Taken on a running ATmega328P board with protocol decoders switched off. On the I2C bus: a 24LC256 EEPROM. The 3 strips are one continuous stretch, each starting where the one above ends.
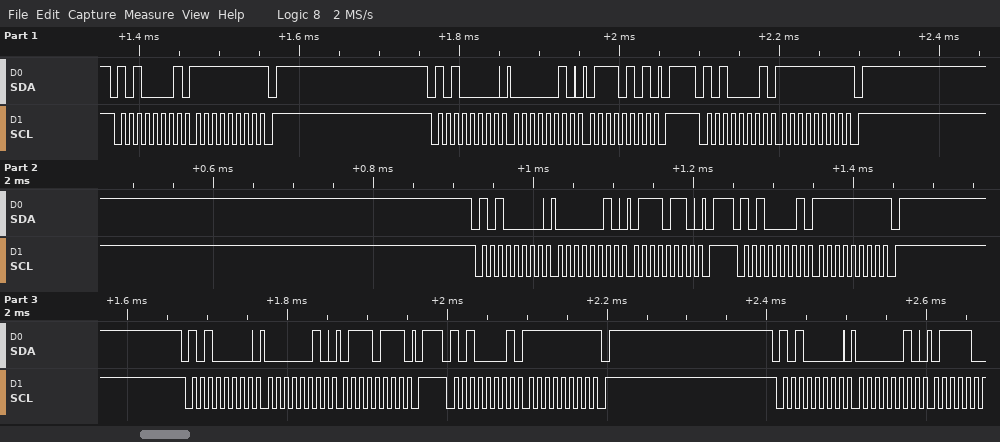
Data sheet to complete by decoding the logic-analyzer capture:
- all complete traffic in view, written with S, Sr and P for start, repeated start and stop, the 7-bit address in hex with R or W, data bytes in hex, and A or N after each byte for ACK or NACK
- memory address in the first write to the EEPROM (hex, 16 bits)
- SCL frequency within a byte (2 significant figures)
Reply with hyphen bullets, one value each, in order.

- S 50R A FF N P S 50W A 02 A 75 A P S 50R A FF N P S 50W A 02 A 76 A P S 50R A FF N P S 50W A 02 A 77 A P S 50R A FF N P S 50W A 02 A
- 0x0275
- 100 kHz
